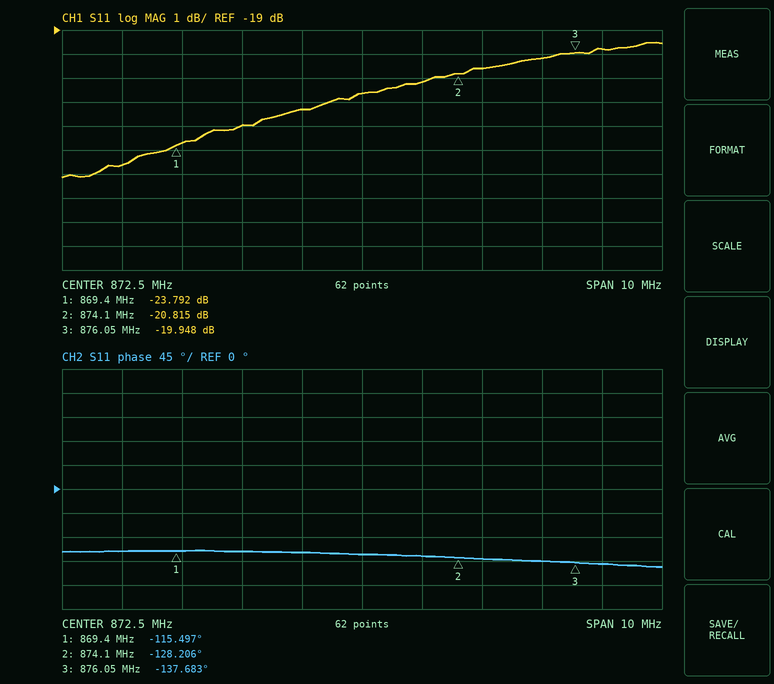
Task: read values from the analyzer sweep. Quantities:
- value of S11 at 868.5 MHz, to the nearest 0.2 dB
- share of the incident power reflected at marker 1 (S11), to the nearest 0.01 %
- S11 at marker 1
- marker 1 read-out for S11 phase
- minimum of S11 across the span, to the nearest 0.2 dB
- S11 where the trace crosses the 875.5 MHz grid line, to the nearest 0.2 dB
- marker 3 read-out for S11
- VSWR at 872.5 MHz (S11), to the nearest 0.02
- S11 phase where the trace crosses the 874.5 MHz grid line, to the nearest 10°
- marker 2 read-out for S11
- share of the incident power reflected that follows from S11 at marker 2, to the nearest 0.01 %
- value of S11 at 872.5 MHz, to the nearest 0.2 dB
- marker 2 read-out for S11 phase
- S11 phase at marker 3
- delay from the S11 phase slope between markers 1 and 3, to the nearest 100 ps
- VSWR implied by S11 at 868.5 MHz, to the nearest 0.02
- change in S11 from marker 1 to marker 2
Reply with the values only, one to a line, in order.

-24.6 dB
0.42 %
-23.792 dB
-115.497°
-25.2 dB
-20.2 dB
-19.948 dB
1.18
-130°
-20.815 dB
0.83 %
-21.6 dB
-128.206°
-137.683°
9.3 ns
1.12
2.977 dB
